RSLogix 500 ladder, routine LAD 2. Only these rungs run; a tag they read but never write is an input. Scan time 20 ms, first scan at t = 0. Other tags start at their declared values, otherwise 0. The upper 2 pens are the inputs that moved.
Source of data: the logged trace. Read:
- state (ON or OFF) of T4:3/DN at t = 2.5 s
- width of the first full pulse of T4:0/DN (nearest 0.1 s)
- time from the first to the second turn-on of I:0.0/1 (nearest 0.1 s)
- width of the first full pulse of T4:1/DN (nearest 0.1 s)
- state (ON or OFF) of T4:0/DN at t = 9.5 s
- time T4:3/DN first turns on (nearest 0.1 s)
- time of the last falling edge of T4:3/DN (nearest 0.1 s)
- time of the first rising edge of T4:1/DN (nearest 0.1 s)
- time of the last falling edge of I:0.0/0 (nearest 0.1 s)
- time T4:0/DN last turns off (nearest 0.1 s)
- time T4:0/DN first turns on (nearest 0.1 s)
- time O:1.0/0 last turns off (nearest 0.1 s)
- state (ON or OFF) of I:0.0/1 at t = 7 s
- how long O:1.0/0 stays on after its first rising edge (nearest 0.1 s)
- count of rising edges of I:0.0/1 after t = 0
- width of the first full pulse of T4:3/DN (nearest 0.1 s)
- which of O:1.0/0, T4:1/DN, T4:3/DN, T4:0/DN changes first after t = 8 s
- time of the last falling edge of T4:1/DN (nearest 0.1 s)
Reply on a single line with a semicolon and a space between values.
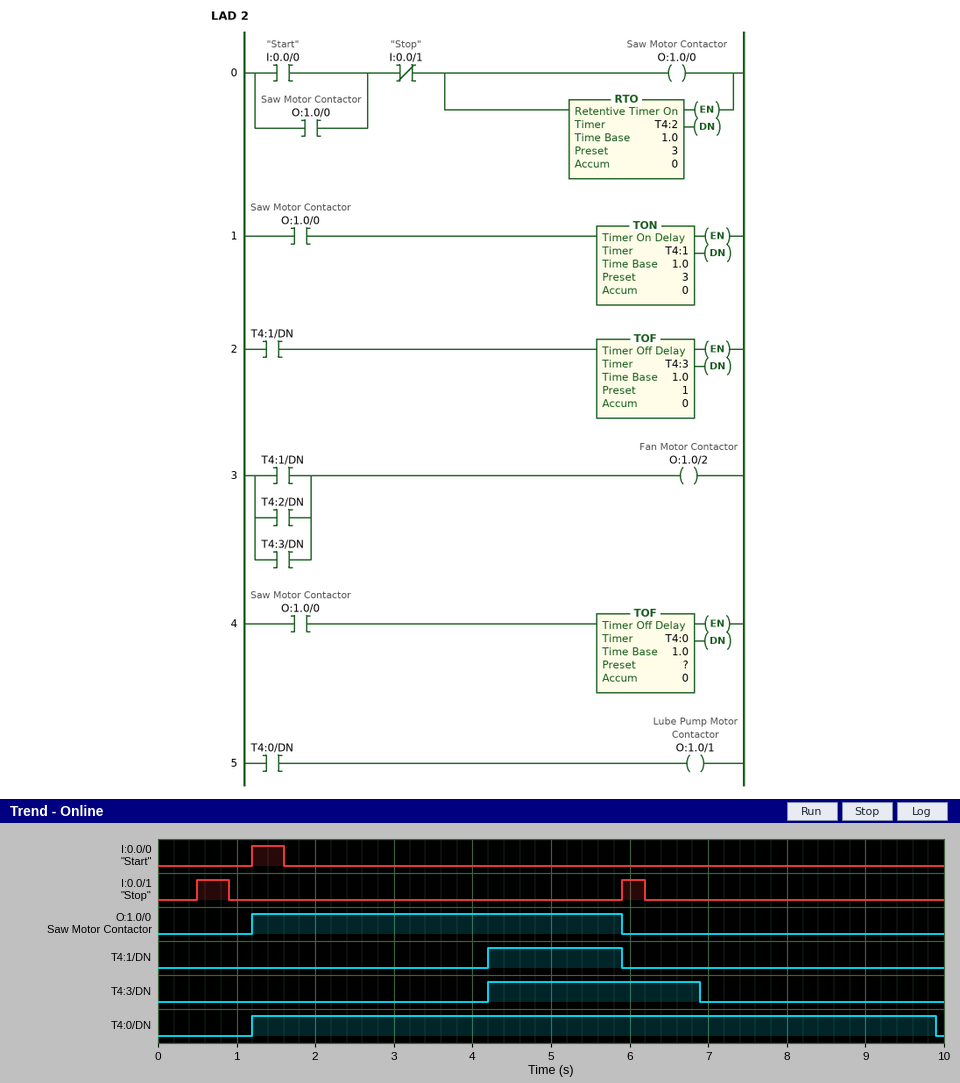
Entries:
OFF; 8.7 s; 5.4 s; 1.7 s; ON; 4.2 s; 6.9 s; 4.2 s; 1.6 s; 9.9 s; 1.2 s; 5.9 s; OFF; 4.7 s; 2; 2.7 s; T4:0/DN; 5.9 s
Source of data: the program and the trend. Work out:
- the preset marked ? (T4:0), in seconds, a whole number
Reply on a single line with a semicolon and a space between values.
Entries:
4 s
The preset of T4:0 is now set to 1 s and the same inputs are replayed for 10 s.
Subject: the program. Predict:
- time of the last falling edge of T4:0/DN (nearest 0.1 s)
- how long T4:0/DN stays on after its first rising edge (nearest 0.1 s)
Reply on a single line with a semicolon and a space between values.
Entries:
6.9 s; 5.7 s
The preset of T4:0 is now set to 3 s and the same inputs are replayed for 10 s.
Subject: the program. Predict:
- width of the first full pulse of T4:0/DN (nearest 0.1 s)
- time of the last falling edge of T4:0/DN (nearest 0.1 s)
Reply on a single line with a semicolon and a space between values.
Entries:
7.7 s; 8.9 s
